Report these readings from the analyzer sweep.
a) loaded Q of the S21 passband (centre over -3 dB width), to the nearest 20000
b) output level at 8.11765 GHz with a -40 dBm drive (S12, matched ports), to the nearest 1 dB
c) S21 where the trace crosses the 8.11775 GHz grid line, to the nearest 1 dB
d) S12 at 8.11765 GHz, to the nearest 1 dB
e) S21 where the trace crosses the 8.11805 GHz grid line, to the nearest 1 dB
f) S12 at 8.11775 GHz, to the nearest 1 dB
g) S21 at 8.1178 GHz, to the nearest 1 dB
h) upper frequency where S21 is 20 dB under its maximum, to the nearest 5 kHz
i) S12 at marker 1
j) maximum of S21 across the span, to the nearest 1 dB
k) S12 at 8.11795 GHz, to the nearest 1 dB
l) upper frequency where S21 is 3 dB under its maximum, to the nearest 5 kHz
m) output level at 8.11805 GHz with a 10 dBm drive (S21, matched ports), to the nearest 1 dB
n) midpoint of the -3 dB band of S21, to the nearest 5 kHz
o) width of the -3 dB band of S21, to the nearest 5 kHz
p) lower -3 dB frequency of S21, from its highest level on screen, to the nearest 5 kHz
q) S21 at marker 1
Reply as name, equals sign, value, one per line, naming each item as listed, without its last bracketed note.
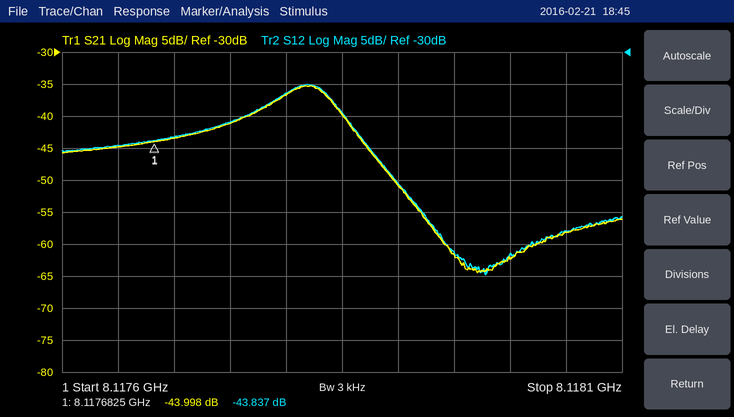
loaded Q of the S21 passband (centre over -3 dB width), to the nearest 20000 = 140000
output level at 8.11765 GHz with a -40 dBm drive (S12, matched ports), to the nearest 1 dB = -85 dBm
S21 where the trace crosses the 8.11775 GHz grid line, to the nearest 1 dB = -41 dB
S12 at 8.11765 GHz, to the nearest 1 dB = -45 dB
S21 where the trace crosses the 8.11805 GHz grid line, to the nearest 1 dB = -58 dB
S12 at 8.11775 GHz, to the nearest 1 dB = -41 dB
S21 at 8.1178 GHz, to the nearest 1 dB = -37 dB
upper frequency where S21 is 20 dB under its maximum, to the nearest 5 kHz = 8.117920 GHz
S12 at marker 1 = -43.837 dB
maximum of S21 across the span, to the nearest 1 dB = -35 dB
S12 at 8.11795 GHz, to the nearest 1 dB = -61 dB
upper frequency where S21 is 3 dB under its maximum, to the nearest 5 kHz = 8.117845 GHz
output level at 8.11805 GHz with a 10 dBm drive (S21, matched ports), to the nearest 1 dB = -48 dBm
midpoint of the -3 dB band of S21, to the nearest 5 kHz = 8.117815 GHz
width of the -3 dB band of S21, to the nearest 5 kHz = 60 kHz
lower -3 dB frequency of S21, from its highest level on screen, to the nearest 5 kHz = 8.117785 GHz
S21 at marker 1 = -43.998 dB
